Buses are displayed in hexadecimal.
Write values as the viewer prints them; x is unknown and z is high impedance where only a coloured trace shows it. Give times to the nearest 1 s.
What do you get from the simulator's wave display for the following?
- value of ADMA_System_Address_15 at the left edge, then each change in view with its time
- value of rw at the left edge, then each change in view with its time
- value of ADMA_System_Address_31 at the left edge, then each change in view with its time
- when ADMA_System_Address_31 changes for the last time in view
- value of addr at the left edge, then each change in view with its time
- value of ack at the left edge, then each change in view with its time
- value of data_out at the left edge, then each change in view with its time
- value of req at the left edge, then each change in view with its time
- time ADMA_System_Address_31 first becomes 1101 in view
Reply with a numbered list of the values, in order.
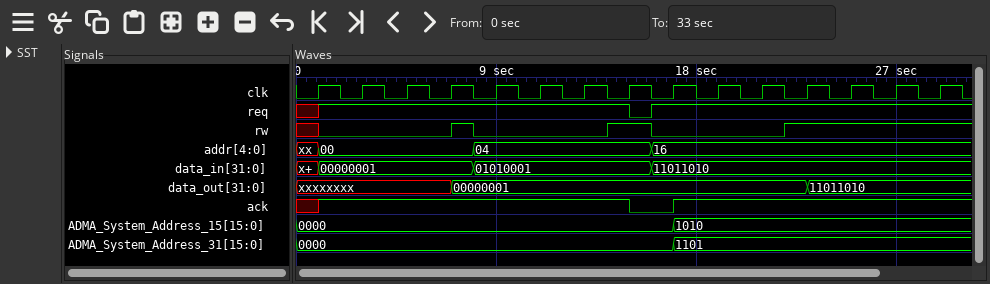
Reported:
1. 0000, 1010 at 17 s
2. x, 0 at 1 s, 1 at 7 s, 0 at 8 s, 1 at 14 s, 0 at 16 s, 1 at 22 s
3. 0000, 1101 at 17 s
4. 17 s
5. xx, 00 at 1 s, 04 at 8 s, 16 at 16 s
6. x, 1 at 1 s, 0 at 15 s, 1 at 17 s
7. xxxxxxxx, 00000001 at 7 s, 11011010 at 23 s
8. x, 1 at 1 s, 0 at 15 s, 1 at 16 s
9. 17 s
